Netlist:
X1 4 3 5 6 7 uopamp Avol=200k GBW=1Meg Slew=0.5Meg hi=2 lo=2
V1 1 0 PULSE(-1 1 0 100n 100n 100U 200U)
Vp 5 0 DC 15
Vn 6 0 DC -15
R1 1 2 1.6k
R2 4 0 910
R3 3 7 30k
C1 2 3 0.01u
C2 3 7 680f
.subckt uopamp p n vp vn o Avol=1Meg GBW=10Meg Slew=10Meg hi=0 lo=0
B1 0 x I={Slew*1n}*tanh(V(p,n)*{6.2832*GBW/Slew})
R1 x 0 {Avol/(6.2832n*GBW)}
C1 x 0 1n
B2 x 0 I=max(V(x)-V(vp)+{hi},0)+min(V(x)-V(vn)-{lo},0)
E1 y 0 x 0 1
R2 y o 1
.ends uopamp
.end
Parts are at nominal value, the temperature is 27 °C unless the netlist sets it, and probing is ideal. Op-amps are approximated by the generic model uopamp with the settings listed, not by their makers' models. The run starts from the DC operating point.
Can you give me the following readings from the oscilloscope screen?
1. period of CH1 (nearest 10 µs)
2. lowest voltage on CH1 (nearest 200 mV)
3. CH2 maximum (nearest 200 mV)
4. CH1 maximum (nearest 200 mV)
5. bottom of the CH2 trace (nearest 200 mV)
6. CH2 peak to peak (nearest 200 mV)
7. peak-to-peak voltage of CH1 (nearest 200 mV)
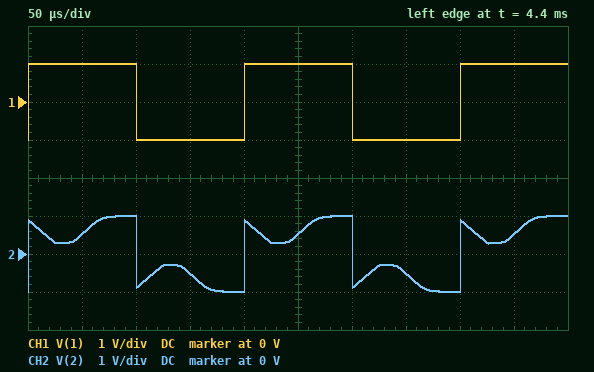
200 µs
-1.0 V
1.0 V
1.0 V
-1.0 V
2.0 V
2.0 V
